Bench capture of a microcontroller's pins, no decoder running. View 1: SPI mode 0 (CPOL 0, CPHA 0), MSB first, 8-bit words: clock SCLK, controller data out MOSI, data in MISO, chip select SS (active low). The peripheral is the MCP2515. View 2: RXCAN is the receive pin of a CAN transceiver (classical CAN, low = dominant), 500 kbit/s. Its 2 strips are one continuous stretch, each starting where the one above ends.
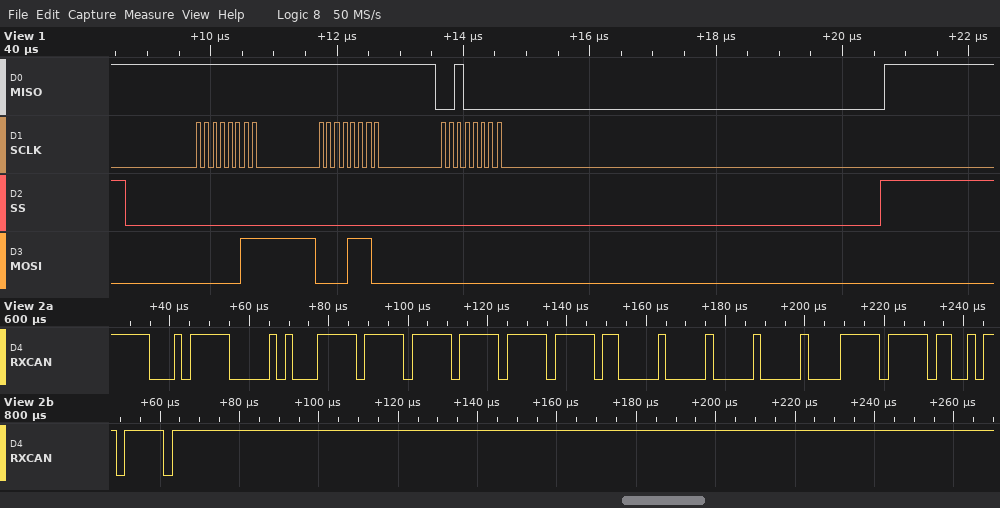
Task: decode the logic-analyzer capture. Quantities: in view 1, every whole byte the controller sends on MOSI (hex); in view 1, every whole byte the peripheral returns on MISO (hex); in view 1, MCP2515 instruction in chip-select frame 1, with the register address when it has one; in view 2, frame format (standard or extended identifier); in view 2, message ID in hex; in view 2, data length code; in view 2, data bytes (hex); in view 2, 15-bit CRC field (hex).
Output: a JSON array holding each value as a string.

["0x03 0x0E 0x00", "0xFF 0xFF 0x20", "READ 0x0E", "standard", "0x17C", "8", "FF FF FF FF 00 00 00 FF", "0x796F"]
